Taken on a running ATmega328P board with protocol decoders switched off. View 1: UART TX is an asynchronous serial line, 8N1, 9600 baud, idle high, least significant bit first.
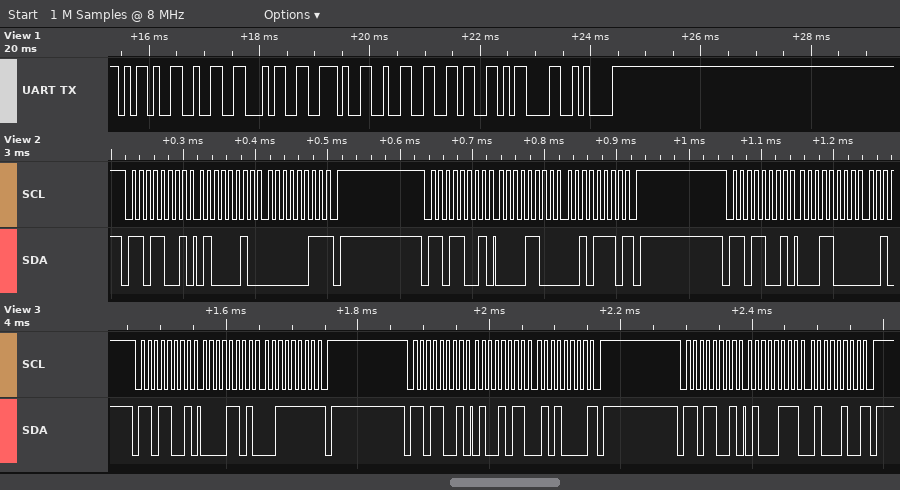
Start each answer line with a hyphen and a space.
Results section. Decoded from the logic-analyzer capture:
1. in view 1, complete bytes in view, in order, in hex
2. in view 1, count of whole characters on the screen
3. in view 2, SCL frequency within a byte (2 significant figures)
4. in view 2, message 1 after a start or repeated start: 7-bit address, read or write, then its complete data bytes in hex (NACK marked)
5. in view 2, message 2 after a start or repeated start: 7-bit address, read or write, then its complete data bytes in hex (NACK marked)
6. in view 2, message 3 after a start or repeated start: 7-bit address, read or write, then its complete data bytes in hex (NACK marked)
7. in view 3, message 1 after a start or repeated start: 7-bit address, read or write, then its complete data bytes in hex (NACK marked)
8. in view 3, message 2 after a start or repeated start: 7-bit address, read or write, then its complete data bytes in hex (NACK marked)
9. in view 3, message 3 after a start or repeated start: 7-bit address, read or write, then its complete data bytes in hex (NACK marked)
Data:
- 2D 32 34 2E 32 36 0D 0A
- 8
- 100 kHz
- 0x6C read: 42 03 NACK
- 0x6C read: 0C 2E NACK
- 0x6C read: 18
- 0x6C read: 0D 3F NACK
- 0x6C read: 4B 50 NACK
- 0x6C read: 47 44 NACK
